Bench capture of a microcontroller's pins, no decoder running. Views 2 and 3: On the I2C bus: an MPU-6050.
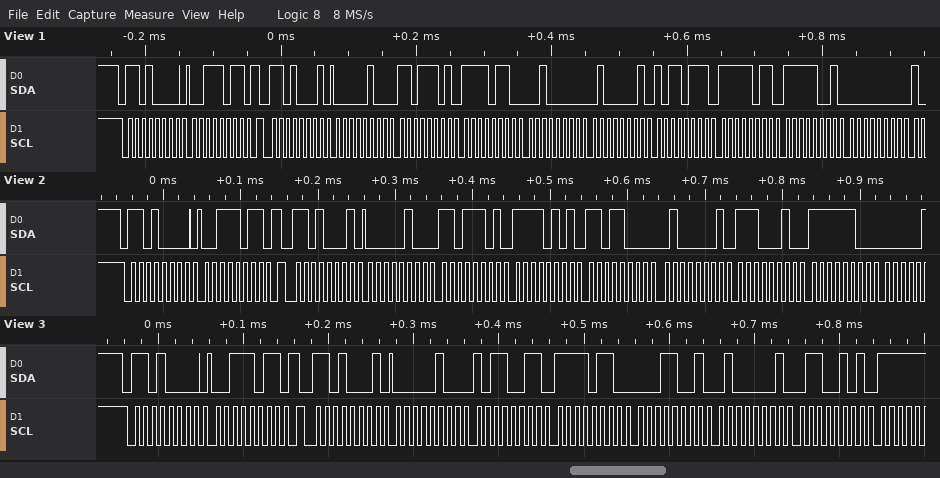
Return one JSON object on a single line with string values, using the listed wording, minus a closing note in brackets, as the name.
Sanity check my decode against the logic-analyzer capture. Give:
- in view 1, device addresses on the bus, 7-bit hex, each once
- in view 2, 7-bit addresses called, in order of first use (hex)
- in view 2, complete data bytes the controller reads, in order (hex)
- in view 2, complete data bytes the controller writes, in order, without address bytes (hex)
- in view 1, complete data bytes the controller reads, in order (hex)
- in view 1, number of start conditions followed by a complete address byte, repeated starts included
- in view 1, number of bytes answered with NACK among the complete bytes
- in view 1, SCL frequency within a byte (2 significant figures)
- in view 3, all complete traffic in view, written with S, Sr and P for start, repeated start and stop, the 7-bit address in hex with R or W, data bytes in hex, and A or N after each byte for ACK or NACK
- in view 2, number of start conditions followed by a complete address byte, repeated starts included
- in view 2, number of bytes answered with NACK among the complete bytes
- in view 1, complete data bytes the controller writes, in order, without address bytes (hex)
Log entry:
{"in view 1, device addresses on the bus, 7-bit hex, each once": "0x68", "in view 2, 7-bit addresses called, in order of first use": "0x68", "in view 2, complete data bytes the controller reads, in order": "04 DD F5 D8 41 E2 FC", "in view 2, complete data bytes the controller writes, in order, without address bytes": "3B", "in view 1, complete data bytes the controller reads, in order": "04 DD F6 20 41 B7 FB F9 00", "in view 1, number of start conditions followed by a complete address byte, repeated starts included": "2", "in view 1, number of bytes answered with NACK among the complete bytes": "0", "in view 1, SCL frequency within a byte": "100 kHz", "in view 3, all complete traffic in view, written with S, Sr and P for start, repeated start and stop, the 7-bit address in hex with R or W, data bytes in hex, and A or N after each byte for ACK or NACK": "S 68W A 3B A Sr 68R A 04 A B3 A F6 A 19 A 41 A 65 A", "in view 2, number of start conditions followed by a complete address byte, repeated starts included": "2", "in view 2, number of bytes answered with NACK among the complete bytes": "0", "in view 1, complete data bytes the controller writes, in order, without address bytes": "3B"}
